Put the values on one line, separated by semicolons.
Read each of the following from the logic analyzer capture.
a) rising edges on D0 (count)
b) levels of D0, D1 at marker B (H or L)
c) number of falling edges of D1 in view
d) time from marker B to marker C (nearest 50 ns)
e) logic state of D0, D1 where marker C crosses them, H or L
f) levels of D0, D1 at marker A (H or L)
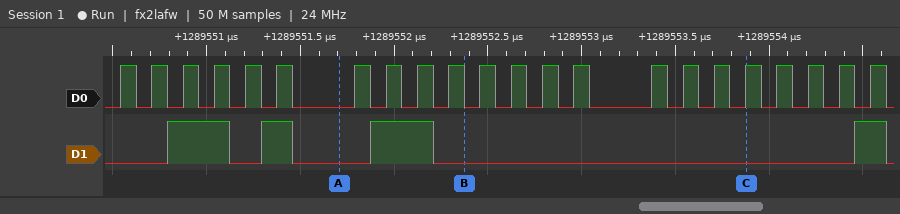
22; D0=L, D1=L; 4; 1500 ns; D0=H, D1=L; D0=L, D1=L
